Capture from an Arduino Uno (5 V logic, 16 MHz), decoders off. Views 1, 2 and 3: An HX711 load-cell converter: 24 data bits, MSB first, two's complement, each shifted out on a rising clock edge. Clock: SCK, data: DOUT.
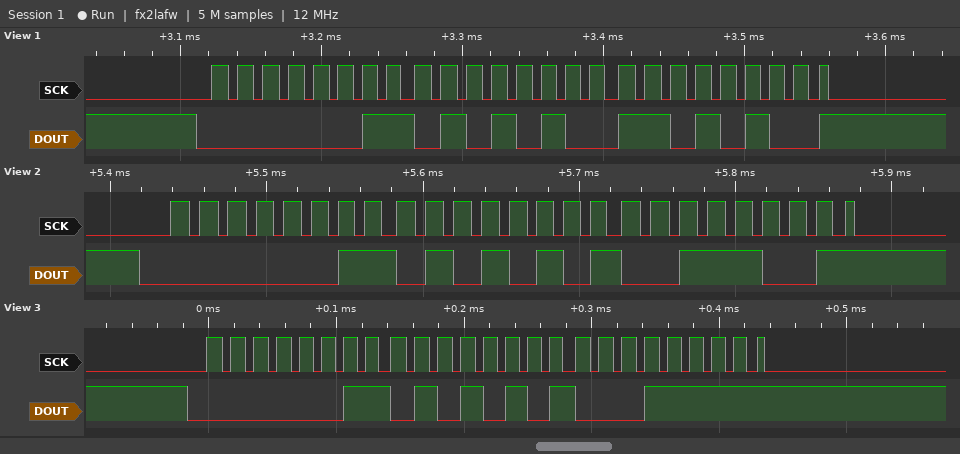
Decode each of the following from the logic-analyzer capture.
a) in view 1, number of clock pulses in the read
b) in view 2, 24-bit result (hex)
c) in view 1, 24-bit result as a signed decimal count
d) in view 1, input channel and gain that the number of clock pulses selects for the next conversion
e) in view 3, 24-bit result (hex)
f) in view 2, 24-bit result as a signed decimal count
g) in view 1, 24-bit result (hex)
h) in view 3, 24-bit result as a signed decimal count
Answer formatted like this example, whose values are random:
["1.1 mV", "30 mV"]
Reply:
["25", "0x035539", "218324", "channel A, gain 128", "0x03551F", "218425", "0x0354D4", "218399"]
